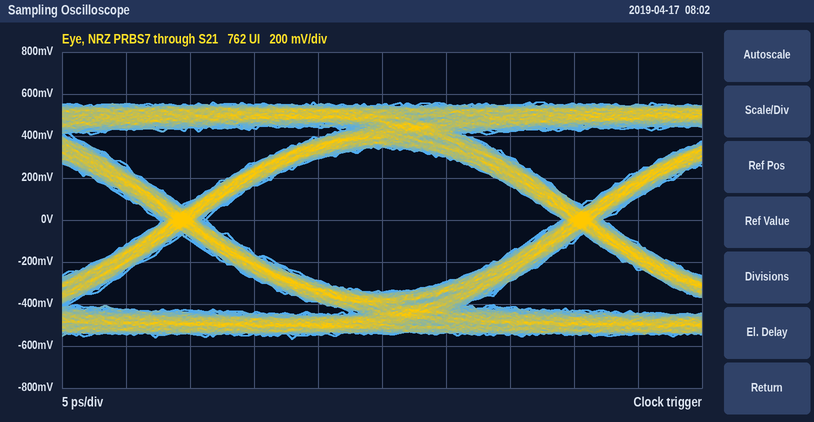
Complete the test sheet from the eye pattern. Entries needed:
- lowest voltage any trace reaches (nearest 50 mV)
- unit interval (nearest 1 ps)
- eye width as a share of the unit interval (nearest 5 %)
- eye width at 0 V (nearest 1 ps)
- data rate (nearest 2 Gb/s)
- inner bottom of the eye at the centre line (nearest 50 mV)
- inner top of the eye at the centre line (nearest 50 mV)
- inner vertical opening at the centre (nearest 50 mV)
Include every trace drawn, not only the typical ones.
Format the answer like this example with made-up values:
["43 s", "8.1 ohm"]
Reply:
["-550 mV", "31 ps", "90 %", "28 ps", "32 Gb/s", "-350 mV", "350 mV", "700 mV"]
